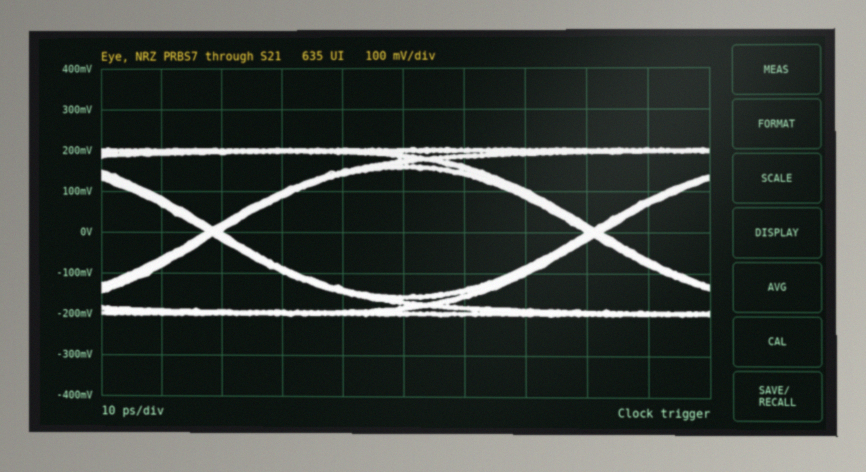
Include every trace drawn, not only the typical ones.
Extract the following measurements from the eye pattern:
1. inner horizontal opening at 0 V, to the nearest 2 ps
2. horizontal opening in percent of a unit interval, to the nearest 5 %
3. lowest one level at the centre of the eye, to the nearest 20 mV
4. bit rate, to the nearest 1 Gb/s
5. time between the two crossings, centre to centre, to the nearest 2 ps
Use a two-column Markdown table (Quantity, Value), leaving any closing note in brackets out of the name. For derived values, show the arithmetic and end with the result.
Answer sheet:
| Quantity | Value |
|---|---|
| inner horizontal opening at 0 V, to the nearest 2 ps | 60 ps |
| horizontal opening in percent of a unit interval, to the nearest 5 % | 60 ps / 62 ps ≈ 96.8 %, so 95 % to the nearest 5 % |
| lowest one level at the centre of the eye, to the nearest 20 mV | 160 mV |
| bit rate, to the nearest 1 Gb/s | 16 Gb/s |
| time between the two crossings, centre to centre, to the nearest 2 ps | 62 ps |
